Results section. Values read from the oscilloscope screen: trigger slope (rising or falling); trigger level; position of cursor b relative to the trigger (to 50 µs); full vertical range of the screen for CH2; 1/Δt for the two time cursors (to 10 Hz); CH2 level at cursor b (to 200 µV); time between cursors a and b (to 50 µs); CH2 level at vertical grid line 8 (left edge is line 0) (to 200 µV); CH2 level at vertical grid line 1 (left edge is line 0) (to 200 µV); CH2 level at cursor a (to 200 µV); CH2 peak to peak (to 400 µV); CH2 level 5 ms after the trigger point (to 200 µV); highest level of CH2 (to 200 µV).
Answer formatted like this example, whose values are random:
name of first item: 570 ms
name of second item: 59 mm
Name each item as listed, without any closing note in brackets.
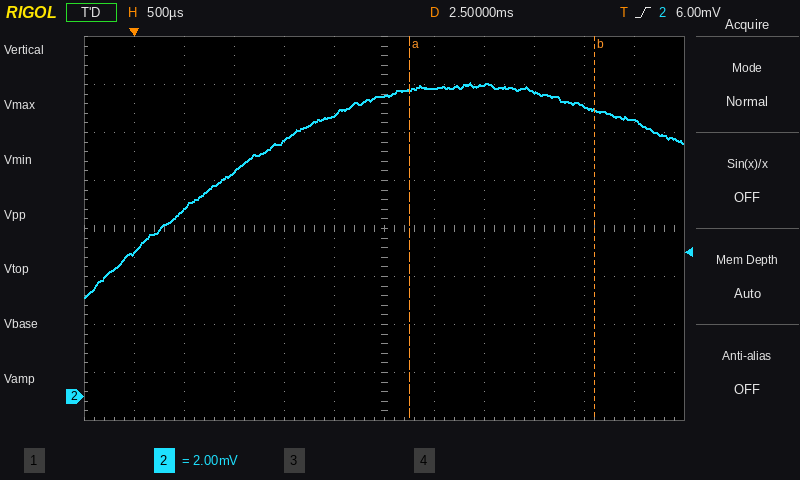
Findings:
trigger slope: rising
trigger level: 6.00 mV
position of cursor b relative to the trigger: +4.60 ms
full vertical range of the screen for CH2: 16 mV
1/Δt for the two time cursors: 540 Hz
CH2 level at cursor b: 12.0 mV
time between cursors a and b: 1.85 ms
CH2 level at vertical grid line 8 (left edge is line 0): 13.0 mV
CH2 level at vertical grid line 1 (left edge is line 0): 6.0 mV
CH2 level at cursor a: 12.8 mV
CH2 peak to peak: 8.8 mV
CH2 level 5 ms after the trigger point: 11.6 mV
highest level of CH2: 13.0 mV
